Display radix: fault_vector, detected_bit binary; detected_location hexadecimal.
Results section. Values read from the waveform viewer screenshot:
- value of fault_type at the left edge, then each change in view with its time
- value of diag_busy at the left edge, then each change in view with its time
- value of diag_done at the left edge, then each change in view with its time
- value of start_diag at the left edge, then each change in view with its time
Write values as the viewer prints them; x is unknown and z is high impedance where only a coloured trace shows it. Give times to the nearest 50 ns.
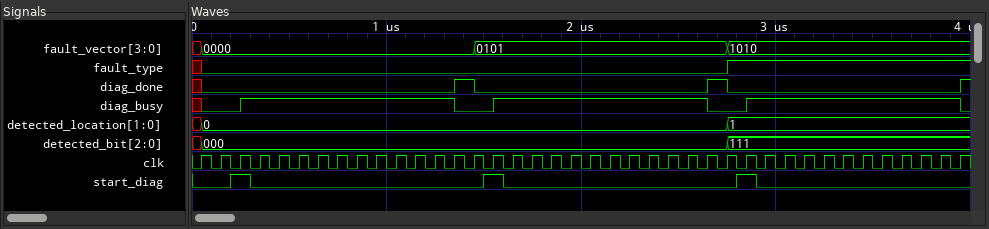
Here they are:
x, 0 at 50 ns, 1 at 2750 ns
x, 0 at 50 ns, 1 at 250 ns, 0 at 1350 ns, 1 at 1550 ns, 0 at 2650 ns, 1 at 2850 ns, 0 at 3950 ns
x, 0 at 50 ns, 1 at 1350 ns, 0 at 1450 ns, 1 at 2650 ns, 0 at 2750 ns, 1 at 3950 ns
0, 1 at 200 ns, 0 at 300 ns, 1 at 1500 ns, 0 at 1600 ns, 1 at 2800 ns, 0 at 2900 ns
